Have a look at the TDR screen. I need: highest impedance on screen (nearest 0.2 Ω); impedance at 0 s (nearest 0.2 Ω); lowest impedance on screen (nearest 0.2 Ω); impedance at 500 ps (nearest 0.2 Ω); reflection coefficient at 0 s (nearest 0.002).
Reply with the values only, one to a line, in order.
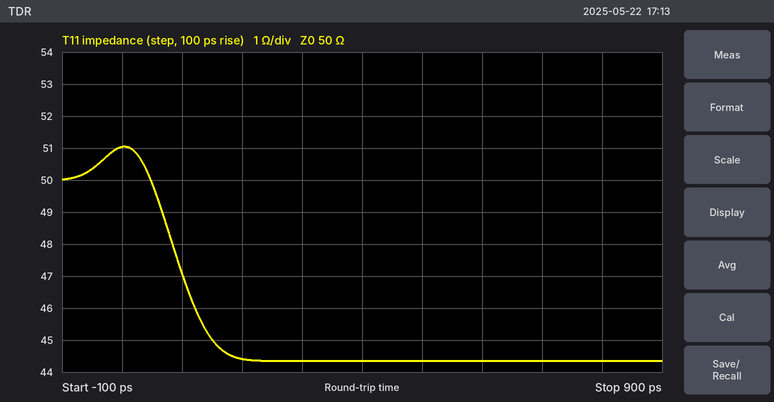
51.0 Ω
51.0 Ω
44.4 Ω
44.4 Ω
+0.010
